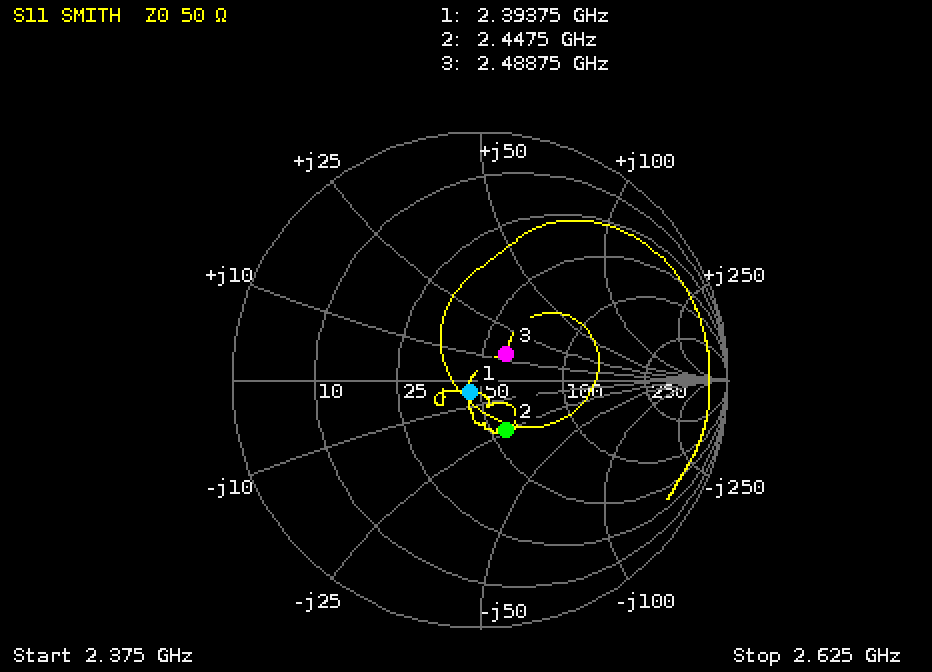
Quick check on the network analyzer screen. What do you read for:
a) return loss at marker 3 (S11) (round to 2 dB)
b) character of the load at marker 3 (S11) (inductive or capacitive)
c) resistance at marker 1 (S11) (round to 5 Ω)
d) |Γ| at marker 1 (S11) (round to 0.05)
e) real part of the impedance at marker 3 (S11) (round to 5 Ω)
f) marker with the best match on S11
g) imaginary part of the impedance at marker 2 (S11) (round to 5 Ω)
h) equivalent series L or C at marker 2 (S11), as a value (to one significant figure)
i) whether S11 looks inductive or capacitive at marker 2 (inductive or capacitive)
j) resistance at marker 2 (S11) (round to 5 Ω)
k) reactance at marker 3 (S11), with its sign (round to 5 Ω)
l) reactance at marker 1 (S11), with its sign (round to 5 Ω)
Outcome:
16 dB
inductive
45 Ω
0.05
60 Ω
marker 1
-25 Ω
3 pF
capacitive
55 Ω
+15 Ω
-5 Ω
